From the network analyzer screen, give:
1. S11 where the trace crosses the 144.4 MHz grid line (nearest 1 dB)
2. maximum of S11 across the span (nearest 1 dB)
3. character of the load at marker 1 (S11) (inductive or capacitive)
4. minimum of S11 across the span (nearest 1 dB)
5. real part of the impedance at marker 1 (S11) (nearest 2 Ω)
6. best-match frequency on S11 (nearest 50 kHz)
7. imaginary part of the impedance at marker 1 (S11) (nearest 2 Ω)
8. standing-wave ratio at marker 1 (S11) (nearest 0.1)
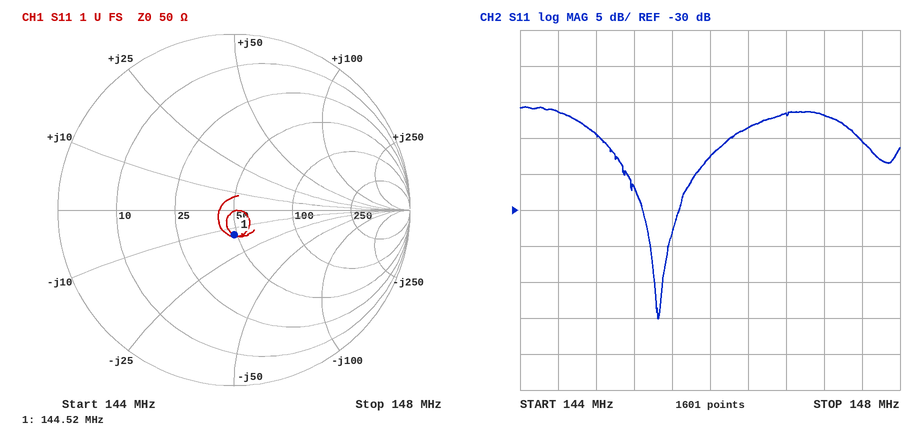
-16 dB
-16 dB
capacitive
-45 dB
48 Ω
145.45 MHz
-14 Ω
1.3
